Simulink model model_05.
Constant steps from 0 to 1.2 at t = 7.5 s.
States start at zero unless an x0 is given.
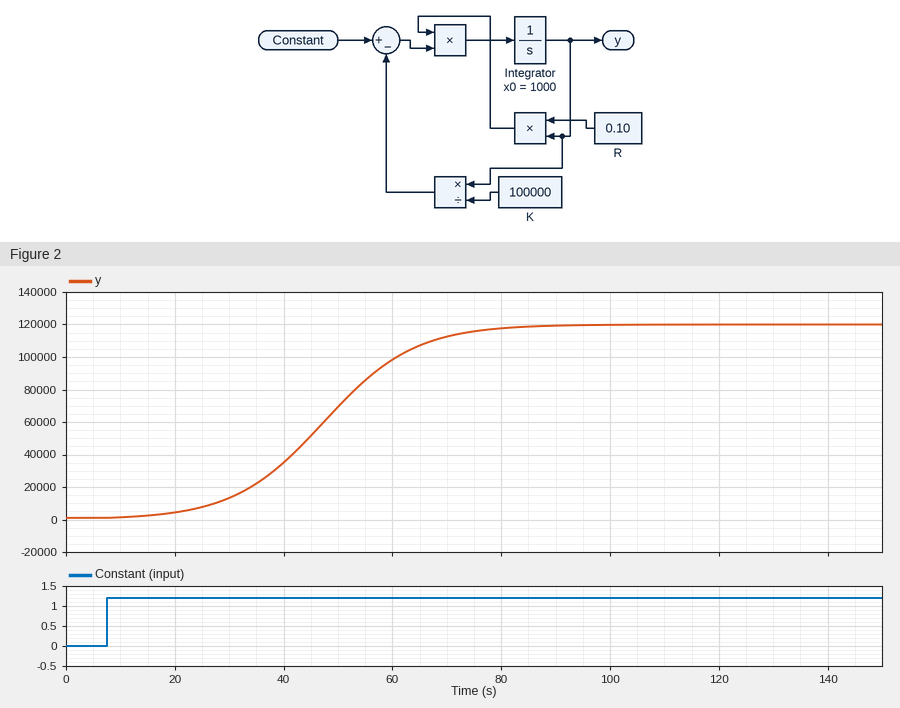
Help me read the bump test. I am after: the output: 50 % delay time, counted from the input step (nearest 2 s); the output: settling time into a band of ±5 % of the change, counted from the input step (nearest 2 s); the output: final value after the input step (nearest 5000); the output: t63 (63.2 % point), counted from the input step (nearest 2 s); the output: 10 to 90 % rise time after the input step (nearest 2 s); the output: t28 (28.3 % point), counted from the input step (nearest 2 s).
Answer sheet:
40 s
64 s
120000
44 s
36 s
32 s
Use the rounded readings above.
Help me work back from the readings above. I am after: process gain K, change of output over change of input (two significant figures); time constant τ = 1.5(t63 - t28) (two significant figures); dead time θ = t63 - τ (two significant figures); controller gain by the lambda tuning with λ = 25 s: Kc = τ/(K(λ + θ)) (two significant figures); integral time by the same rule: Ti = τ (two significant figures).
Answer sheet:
100000
18 s
26 s
0.0000035
18 s
